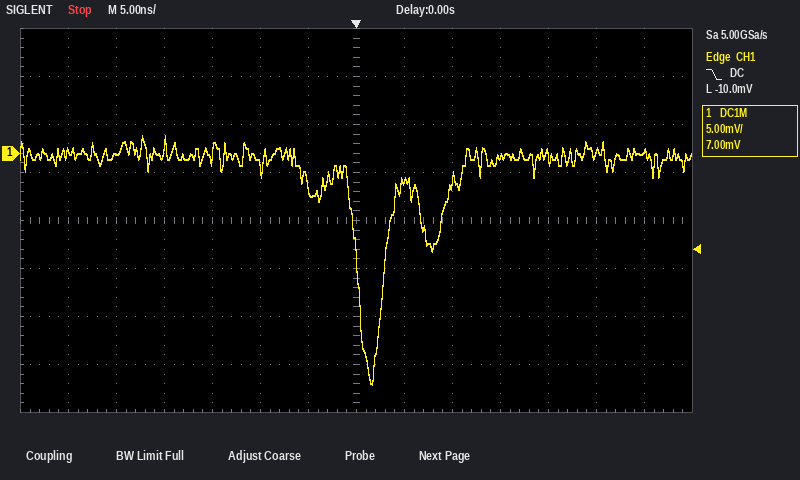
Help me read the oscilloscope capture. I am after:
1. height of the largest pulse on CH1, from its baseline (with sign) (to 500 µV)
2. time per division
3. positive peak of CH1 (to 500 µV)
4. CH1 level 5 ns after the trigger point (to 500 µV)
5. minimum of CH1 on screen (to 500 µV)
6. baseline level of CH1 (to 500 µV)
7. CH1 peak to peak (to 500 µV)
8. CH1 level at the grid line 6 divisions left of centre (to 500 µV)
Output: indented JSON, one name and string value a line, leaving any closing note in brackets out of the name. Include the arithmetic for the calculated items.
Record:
{
  "height of the largest pulse on CH1, from its baseline (with sign)": "-24.0 mV − (-500 µV) = -23.5 mV",
  "time per division": "5 ns",
  "positive peak of CH1": "2.0 mV",
  "CH1 level 5 ns after the trigger point": "-3.0 mV",
  "minimum of CH1 on screen": "-24.0 mV",
  "baseline level of CH1": "-500 µV",
  "CH1 peak to peak": "2.0 mV − (-24.0 mV) = 26.0 mV",
  "CH1 level at the grid line 6 divisions left of centre": "0.0 mV"
}
